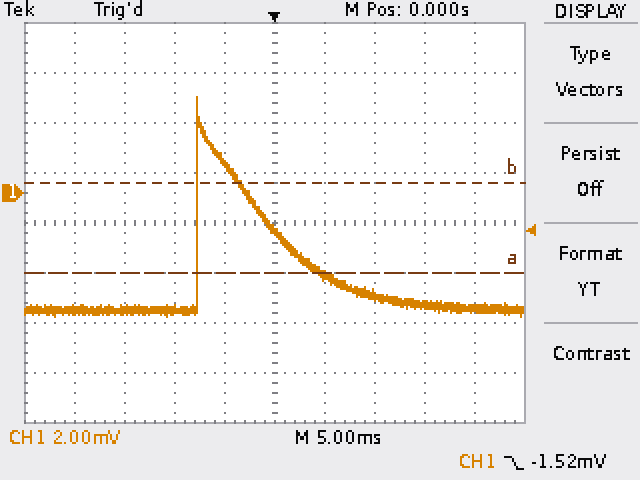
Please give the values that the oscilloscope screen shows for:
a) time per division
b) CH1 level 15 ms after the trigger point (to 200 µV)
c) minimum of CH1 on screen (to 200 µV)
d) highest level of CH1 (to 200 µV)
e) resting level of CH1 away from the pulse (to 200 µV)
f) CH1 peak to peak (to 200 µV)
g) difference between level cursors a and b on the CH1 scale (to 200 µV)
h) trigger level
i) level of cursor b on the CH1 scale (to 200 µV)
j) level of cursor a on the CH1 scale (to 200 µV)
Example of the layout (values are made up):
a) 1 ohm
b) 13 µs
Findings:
a) 5 ms
b) -4.4 mV
c) -5.0 mV
d) 3.8 mV
e) -4.6 mV
f) 8.8 mV
g) 3.6 mV
h) -1.52 mV
i) 400 µV
j) -3.2 mV
